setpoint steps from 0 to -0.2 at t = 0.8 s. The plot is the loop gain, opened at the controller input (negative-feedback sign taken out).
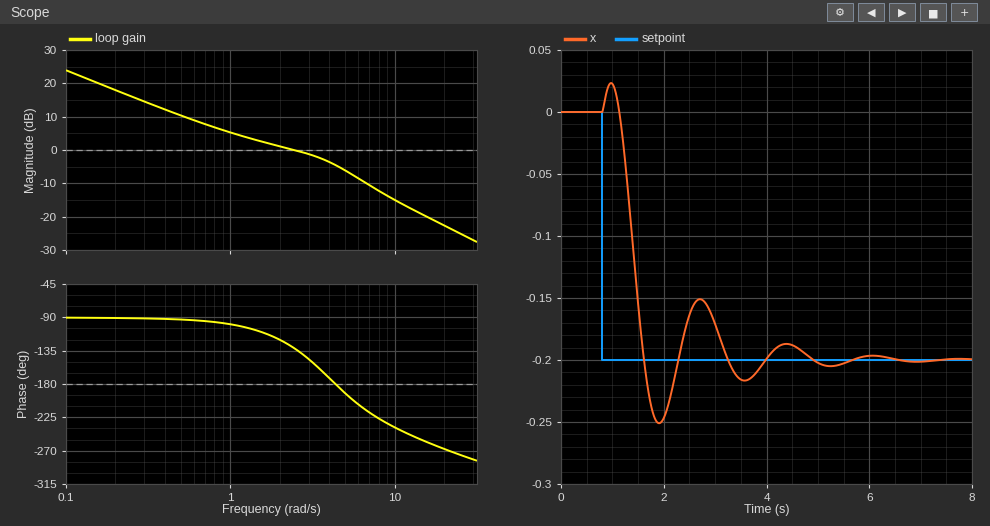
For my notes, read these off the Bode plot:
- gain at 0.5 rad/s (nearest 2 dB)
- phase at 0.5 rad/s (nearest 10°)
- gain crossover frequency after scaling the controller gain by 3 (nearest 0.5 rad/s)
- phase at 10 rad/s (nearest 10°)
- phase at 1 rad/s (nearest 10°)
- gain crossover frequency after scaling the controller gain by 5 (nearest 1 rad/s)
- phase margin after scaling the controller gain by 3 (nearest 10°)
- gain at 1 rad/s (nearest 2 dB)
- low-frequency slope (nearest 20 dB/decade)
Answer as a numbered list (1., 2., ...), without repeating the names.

1. 10 dB
2. -90°
3. 6.5 rad/s
4. -240°
5. -100°
6. 9 rad/s
7. -30°
8. 6 dB
9. -20 dB/decade
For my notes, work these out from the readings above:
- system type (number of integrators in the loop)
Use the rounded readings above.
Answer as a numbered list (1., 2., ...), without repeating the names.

1. 1
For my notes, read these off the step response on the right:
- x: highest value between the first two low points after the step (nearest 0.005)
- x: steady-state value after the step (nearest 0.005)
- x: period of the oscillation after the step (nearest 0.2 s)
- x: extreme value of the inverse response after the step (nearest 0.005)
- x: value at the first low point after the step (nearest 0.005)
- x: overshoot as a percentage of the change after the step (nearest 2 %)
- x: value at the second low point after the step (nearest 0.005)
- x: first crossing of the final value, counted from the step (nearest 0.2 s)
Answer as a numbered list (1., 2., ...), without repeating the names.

1. -0.150
2. -0.200
3. 1.6 s
4. 0.025
5. -0.250
6. 26 %
7. -0.215
8. 0.8 s
